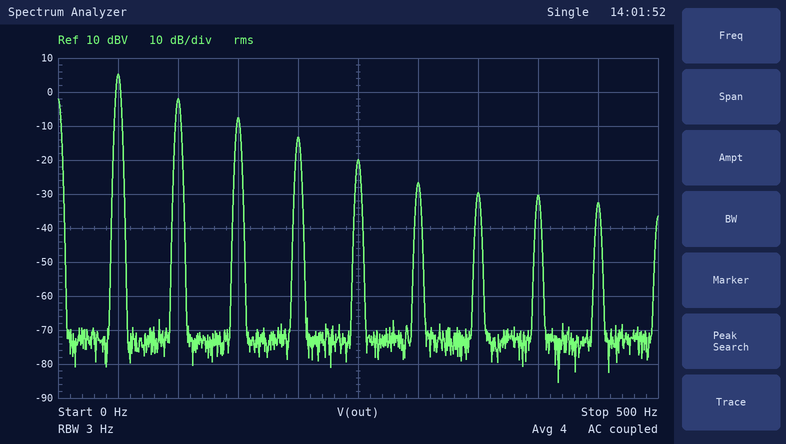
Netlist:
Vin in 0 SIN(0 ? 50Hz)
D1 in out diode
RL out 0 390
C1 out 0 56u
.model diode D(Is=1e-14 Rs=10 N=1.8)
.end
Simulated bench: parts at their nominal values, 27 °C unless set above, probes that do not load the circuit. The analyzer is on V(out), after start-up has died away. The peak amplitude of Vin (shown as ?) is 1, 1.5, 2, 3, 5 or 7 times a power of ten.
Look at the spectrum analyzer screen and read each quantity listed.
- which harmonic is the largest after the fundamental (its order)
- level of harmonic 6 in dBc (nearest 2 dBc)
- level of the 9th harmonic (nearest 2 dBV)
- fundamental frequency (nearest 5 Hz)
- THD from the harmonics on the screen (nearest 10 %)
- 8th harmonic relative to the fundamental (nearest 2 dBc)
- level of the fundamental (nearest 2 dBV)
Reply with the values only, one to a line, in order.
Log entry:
2
-32 dBc
-32 dBV
50 Hz
50 %
-36 dBc
6 dBV
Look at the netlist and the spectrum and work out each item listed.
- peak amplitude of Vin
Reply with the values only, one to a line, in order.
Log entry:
15 V
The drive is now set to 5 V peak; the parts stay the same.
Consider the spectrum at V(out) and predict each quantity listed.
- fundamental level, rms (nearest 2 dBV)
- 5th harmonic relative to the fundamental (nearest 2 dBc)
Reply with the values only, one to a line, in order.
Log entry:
-6 dBV
-24 dBc
